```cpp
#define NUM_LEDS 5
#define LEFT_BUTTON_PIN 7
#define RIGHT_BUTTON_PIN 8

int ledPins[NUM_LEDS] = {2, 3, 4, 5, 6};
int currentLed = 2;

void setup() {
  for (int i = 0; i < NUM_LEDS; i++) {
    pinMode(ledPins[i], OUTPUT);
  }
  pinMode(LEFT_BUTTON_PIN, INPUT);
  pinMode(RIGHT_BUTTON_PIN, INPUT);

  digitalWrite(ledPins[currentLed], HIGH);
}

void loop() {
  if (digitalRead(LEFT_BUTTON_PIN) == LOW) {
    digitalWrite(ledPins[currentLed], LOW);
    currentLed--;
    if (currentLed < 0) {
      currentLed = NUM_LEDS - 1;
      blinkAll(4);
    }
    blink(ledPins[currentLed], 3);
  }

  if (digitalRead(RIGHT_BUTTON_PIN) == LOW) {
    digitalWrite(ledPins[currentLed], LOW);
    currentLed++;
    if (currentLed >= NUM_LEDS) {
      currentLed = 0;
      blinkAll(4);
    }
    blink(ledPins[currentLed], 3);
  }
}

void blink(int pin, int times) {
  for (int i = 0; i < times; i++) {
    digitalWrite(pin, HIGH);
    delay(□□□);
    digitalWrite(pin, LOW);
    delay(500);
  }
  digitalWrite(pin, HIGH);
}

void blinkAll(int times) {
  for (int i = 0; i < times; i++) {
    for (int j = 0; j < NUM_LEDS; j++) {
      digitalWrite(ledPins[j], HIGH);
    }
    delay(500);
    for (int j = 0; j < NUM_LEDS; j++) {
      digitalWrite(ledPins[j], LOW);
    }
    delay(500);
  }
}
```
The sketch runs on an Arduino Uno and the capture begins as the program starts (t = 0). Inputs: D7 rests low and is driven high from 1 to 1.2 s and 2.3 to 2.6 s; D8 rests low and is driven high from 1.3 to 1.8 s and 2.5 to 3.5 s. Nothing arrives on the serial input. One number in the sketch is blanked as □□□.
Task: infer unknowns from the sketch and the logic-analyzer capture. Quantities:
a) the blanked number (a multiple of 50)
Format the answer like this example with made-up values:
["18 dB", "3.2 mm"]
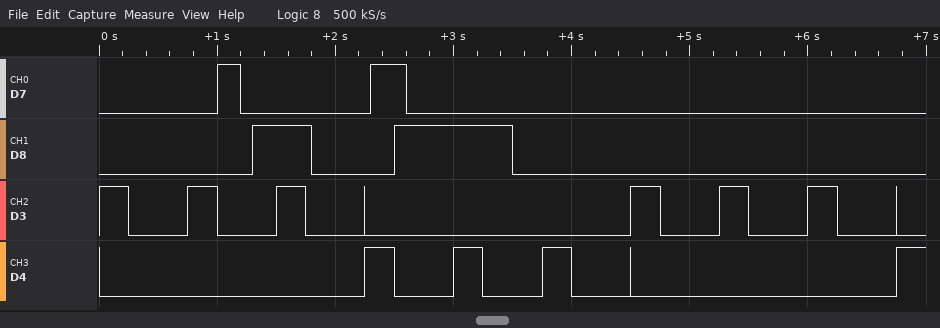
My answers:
["250"]
